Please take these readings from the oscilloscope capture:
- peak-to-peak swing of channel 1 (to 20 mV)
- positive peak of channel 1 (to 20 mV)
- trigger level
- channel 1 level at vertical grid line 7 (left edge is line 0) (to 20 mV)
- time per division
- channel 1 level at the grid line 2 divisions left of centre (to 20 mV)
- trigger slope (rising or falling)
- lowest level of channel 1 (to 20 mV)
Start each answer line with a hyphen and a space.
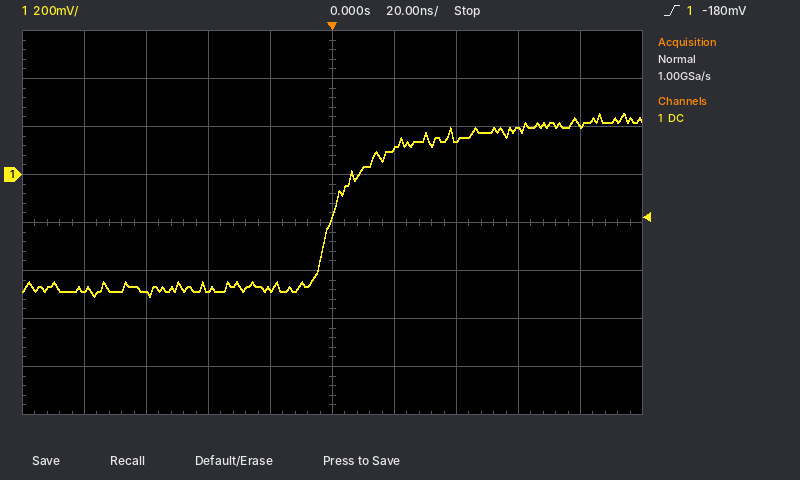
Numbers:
- 760 mV
- 260 mV
- -180 mV
- 140 mV
- 20 ns
- -480 mV
- rising
- -500 mV
